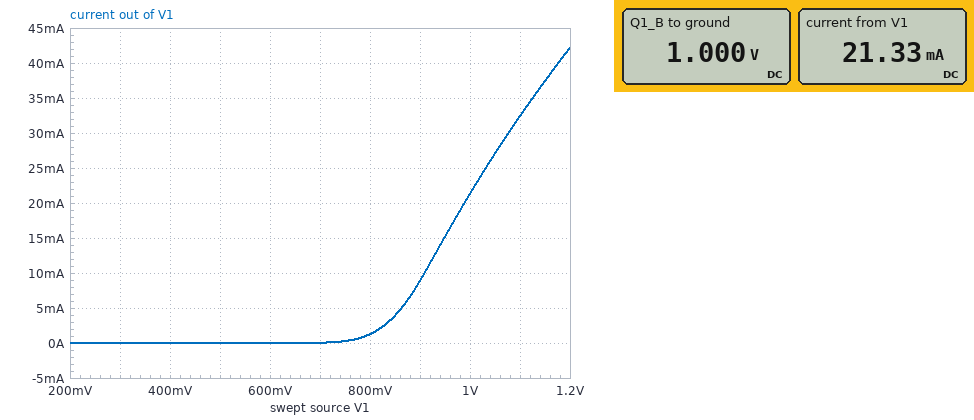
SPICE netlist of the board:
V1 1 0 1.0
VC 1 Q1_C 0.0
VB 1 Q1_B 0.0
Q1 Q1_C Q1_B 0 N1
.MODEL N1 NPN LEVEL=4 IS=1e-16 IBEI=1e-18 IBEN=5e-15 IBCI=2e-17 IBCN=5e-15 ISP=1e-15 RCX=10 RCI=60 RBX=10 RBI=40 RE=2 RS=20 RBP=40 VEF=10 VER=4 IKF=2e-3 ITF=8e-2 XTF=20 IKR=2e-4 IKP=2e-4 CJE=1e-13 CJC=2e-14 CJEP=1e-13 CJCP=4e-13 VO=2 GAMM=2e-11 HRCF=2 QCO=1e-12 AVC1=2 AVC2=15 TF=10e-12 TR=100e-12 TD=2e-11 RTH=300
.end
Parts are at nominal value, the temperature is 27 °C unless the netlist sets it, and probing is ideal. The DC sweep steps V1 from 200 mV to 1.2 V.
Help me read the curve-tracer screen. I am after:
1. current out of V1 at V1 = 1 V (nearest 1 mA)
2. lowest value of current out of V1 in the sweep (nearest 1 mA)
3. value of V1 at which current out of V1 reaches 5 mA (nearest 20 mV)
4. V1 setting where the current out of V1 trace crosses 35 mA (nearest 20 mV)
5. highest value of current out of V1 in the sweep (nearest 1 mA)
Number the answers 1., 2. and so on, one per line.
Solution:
1. 21 mA
2. 0 A
3. 860 mV
4. 1.12 V
5. 42 mA
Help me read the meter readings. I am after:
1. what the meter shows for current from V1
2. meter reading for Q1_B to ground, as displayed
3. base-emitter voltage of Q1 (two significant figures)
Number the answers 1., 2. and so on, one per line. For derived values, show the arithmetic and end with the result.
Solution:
1. 21.33 mA
2. 1.000 V
3. 1 V = 1.0 V
